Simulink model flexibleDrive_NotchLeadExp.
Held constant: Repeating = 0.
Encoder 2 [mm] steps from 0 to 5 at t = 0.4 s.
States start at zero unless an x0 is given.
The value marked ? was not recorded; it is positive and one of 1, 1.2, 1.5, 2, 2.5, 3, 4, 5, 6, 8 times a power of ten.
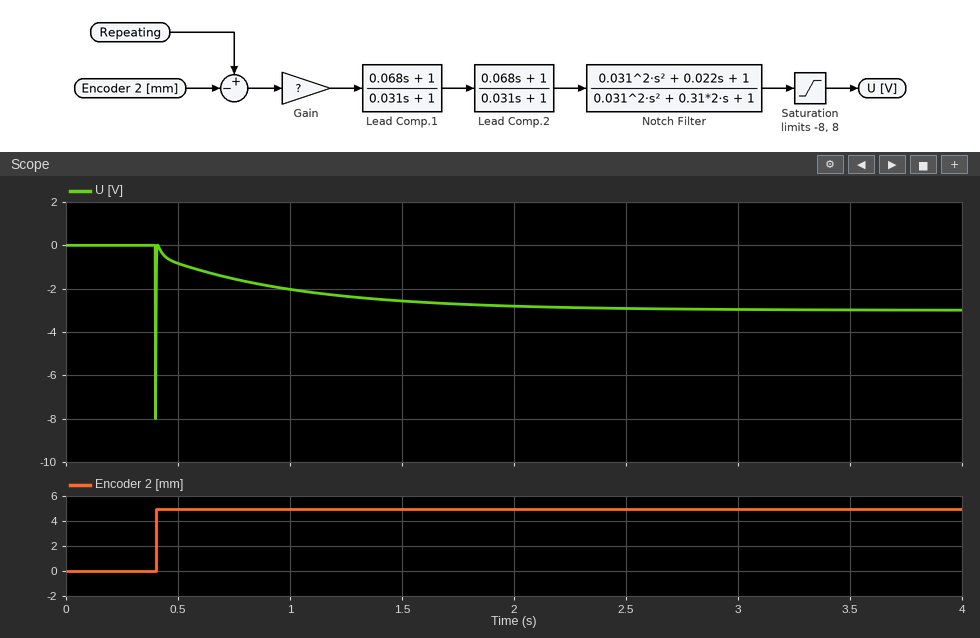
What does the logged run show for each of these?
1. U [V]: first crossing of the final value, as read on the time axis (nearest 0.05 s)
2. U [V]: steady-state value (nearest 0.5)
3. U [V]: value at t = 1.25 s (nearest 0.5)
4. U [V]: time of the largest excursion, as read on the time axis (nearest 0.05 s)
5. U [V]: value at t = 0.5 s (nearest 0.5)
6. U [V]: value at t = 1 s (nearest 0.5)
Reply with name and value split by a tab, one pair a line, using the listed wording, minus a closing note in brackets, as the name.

U [V]: first crossing of the final value, as read on the time axis	0.40 s
U [V]: steady-state value	-3.0
U [V]: value at t = 1.25 s	-2.5
U [V]: time of the largest excursion, as read on the time axis	0.40 s
U [V]: value at t = 0.5 s	-1.0
U [V]: value at t = 1 s	-2.0
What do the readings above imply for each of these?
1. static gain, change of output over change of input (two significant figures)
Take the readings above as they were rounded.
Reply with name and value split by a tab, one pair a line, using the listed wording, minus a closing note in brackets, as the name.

static gain, change of output over change of input	-0.60
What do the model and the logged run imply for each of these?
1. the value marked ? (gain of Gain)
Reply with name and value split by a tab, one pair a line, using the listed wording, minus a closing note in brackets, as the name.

the value marked ?	0.6
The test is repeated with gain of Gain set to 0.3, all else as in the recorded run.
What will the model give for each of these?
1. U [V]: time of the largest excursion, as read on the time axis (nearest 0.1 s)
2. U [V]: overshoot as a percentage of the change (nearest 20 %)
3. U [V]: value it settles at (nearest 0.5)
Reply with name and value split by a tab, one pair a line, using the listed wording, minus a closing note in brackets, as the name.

U [V]: time of the largest excursion, as read on the time axis	0.4 s
U [V]: overshoot as a percentage of the change	380 %
U [V]: value it settles at	-1.5
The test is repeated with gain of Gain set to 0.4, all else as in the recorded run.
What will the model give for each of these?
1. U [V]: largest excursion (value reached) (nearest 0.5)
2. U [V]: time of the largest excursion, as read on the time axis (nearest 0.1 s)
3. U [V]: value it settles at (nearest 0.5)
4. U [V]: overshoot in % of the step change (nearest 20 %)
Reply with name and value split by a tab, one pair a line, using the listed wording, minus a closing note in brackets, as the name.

U [V]: largest excursion (value reached)	-8.0
U [V]: time of the largest excursion, as read on the time axis	0.4 s
U [V]: value it settles at	-2.0
U [V]: overshoot in % of the step change	300 %
